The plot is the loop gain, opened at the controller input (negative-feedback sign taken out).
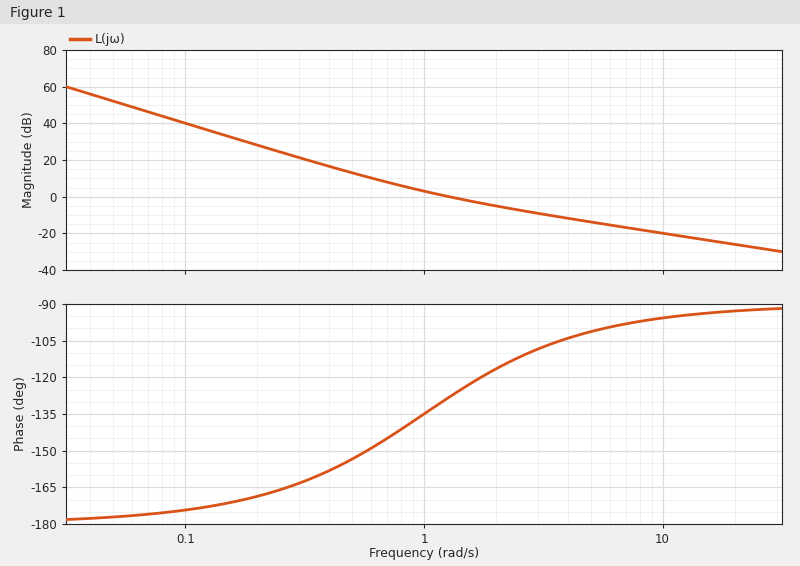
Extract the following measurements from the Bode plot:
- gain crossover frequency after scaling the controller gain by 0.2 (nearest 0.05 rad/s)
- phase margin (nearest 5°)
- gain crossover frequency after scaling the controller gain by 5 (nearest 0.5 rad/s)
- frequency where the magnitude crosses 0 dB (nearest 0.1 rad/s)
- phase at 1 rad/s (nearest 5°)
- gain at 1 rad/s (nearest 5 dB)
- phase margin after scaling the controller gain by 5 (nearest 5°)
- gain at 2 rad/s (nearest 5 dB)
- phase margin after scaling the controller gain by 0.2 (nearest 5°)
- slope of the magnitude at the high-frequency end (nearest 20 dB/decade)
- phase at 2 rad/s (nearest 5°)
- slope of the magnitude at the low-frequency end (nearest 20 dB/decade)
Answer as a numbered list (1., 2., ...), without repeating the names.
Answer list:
1. 0.45 rad/s
2. 50°
3. 5.0 rad/s
4. 1.3 rad/s
5. -135°
6. 5 dB
7. 80°
8. -5 dB
9. 25°
10. -20 dB/decade
11. -115°
12. -40 dB/decade
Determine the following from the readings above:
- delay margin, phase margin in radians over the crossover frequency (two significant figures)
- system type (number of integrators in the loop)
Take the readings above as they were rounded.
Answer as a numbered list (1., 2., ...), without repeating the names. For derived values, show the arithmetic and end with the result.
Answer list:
1. 50 × π / 180 / 1.3 = 0.67 s
2. 2
